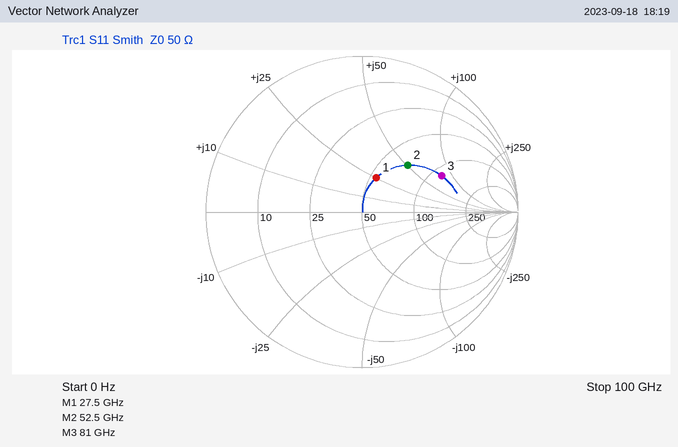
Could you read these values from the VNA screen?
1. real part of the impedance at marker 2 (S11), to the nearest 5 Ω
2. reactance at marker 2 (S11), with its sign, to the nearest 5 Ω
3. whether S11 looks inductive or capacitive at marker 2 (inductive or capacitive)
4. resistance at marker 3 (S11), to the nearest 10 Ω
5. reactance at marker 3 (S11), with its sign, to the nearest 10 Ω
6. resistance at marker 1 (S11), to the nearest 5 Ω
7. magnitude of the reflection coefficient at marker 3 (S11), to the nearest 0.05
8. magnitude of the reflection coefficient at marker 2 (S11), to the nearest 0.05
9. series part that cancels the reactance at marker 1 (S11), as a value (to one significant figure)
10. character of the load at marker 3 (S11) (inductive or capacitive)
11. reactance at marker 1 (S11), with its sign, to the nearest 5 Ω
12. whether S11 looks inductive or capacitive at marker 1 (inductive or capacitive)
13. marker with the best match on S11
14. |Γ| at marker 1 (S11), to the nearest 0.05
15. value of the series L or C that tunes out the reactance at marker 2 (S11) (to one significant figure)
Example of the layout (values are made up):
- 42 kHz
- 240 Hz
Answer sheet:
- 70 Ω
- +50 Ω
- inductive
- 120 Ω
- +80 Ω
- 55 Ω
- 0.55
- 0.40
- 200 fF
- inductive
- +25 Ω
- inductive
- marker 1
- 0.25
- 60 fF
